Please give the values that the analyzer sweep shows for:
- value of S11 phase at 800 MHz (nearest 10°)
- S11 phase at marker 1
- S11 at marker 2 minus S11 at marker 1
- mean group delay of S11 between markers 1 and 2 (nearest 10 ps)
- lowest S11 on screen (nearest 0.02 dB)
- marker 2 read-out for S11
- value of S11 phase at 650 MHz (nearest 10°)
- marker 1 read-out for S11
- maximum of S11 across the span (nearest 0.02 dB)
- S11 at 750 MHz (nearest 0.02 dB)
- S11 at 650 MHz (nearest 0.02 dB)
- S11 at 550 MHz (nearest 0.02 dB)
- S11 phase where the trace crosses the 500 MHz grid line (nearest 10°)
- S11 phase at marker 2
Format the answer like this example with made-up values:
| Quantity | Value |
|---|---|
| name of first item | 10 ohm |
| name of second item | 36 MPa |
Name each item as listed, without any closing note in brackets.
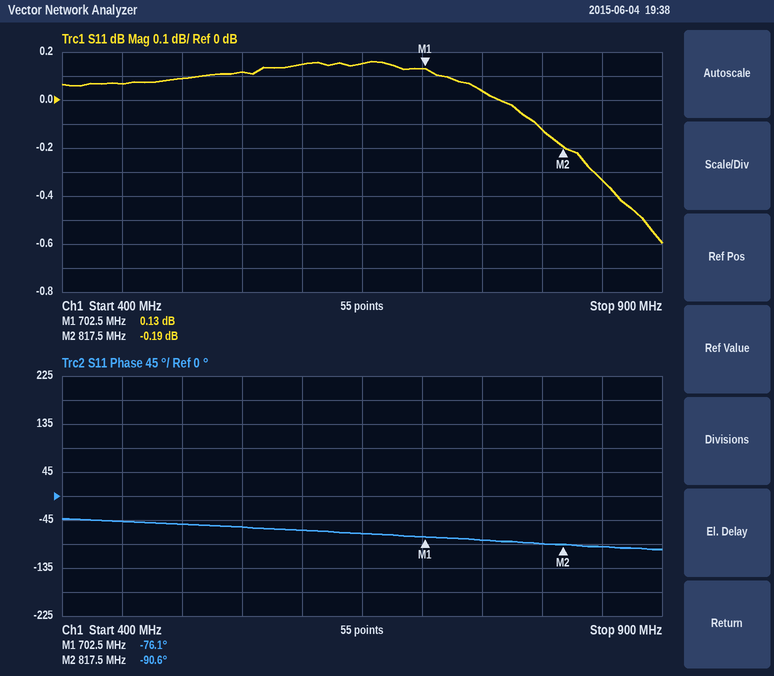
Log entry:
| Quantity | Value |
|---|---|
| value of S11 phase at 800 MHz | -90° |
| S11 phase at marker 1 | -76.1° |
| S11 at marker 2 minus S11 at marker 1 | -0.32 dB |
| mean group delay of S11 between markers 1 and 2 | 350 ps |
| lowest S11 on screen | -0.60 dB |
| marker 2 read-out for S11 | -0.19 dB |
| value of S11 phase at 650 MHz | -70° |
| marker 1 read-out for S11 | 0.13 dB |
| maximum of S11 across the span | 0.16 dB |
| S11 at 750 MHz | 0.04 dB |
| S11 at 650 MHz | 0.16 dB |
| S11 at 550 MHz | 0.12 dB |
| S11 phase where the trace crosses the 500 MHz grid line | -50° |
| S11 phase at marker 2 | -90.6° |
